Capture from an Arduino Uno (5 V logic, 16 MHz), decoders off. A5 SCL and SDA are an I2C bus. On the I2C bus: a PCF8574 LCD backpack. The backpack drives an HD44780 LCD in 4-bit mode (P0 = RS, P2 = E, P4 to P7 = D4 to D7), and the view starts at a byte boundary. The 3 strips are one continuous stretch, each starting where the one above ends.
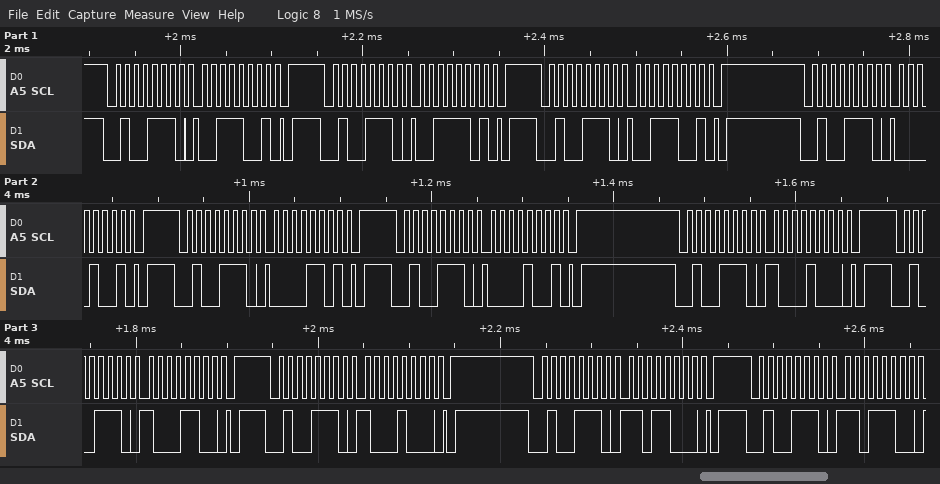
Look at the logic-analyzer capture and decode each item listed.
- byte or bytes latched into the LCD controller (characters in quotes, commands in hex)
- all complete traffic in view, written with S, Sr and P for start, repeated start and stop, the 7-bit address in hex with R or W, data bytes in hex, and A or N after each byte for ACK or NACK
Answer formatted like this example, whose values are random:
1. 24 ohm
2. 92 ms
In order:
1. '0'
2. S 27W A 39 A P S 27W A 3D A P S 27W A 39 A P S 27W A 09 A P S 27W A 0D A P S 27W A 09 A P S 27W A 88 A P S 27W A 8C A P S 27W A 88 A P S 27W A D8 A P S 27W A DC A
